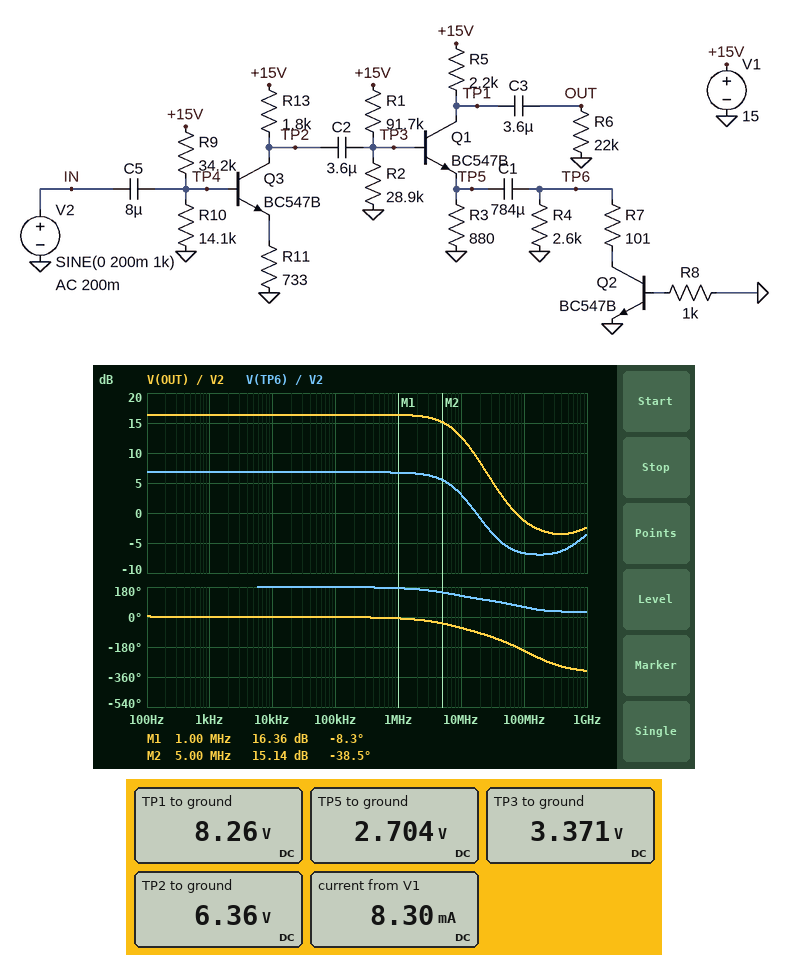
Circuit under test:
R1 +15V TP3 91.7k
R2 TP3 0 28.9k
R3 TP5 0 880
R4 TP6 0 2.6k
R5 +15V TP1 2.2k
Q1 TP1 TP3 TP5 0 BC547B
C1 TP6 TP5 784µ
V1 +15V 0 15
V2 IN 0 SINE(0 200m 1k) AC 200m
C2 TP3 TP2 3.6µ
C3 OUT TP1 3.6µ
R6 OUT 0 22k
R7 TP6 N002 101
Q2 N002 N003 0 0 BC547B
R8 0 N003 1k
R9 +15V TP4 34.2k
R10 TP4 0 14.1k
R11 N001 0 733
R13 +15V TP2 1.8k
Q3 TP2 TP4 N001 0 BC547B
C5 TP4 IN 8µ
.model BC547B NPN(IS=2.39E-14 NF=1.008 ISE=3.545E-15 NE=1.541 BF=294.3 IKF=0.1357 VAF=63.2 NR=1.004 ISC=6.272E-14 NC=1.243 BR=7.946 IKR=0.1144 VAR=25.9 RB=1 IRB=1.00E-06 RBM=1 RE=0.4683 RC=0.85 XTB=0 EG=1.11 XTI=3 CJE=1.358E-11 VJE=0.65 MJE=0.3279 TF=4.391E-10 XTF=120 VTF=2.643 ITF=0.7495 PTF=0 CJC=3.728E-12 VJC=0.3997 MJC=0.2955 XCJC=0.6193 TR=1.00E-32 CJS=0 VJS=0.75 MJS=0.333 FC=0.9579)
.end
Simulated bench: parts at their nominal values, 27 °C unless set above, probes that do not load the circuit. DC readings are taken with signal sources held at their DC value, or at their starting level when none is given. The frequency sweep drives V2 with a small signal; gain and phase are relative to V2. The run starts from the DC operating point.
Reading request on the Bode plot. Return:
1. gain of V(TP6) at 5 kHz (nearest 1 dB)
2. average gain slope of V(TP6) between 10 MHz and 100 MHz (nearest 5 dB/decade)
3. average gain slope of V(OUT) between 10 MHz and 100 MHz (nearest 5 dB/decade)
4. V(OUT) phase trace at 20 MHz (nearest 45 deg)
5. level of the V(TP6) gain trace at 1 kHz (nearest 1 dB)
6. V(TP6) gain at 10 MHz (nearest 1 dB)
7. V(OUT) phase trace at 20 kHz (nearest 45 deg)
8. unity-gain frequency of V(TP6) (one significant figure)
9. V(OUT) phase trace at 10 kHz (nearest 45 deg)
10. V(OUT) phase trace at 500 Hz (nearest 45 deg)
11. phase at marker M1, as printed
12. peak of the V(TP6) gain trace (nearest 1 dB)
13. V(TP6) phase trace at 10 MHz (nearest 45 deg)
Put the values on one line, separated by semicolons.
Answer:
7 dB; -10 dB/decade; -15 dB/decade; -90 deg; 7 dB; 3 dB; 0 deg; 20 MHz; 0 deg; 0 deg; -8.3 deg; 7 dB; 135 deg
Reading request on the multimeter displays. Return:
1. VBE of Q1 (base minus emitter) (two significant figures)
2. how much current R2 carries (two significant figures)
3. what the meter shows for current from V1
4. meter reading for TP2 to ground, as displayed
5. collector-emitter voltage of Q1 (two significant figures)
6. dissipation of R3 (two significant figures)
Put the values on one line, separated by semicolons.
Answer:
670 mV; 120 µA; 8.30 mA; 6.36 V; 5.6 V; 8.3 mW
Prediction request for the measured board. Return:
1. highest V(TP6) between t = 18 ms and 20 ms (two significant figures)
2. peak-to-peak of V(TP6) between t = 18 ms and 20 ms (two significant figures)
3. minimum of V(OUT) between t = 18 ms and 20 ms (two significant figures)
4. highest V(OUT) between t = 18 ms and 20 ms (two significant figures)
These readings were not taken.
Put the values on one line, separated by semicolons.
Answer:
440 mV; 870 mV; -1.3 V; 1.3 V
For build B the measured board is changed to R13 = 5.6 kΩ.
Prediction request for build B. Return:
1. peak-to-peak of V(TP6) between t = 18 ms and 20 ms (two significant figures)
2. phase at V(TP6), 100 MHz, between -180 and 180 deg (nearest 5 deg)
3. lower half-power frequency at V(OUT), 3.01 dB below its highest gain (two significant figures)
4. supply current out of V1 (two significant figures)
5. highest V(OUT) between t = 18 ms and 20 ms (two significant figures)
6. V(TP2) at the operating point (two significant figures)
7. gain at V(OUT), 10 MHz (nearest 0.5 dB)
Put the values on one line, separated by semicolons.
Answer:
510 mV; 0 deg; 37 Hz; 5.9 mA; 330 mV; 1.9 V; 8.0 dB
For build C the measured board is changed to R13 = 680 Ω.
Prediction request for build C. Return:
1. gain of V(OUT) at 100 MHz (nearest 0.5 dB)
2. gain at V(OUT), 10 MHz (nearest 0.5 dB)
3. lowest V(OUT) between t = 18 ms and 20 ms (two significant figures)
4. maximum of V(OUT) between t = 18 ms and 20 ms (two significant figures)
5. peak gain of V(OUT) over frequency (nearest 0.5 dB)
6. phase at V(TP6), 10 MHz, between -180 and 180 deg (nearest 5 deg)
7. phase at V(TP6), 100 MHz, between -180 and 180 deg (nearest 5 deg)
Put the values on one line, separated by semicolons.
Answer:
-3.0 dB; 7.5 dB; -530 mV; 530 mV; 8.5 dB; 150 deg; 75 deg
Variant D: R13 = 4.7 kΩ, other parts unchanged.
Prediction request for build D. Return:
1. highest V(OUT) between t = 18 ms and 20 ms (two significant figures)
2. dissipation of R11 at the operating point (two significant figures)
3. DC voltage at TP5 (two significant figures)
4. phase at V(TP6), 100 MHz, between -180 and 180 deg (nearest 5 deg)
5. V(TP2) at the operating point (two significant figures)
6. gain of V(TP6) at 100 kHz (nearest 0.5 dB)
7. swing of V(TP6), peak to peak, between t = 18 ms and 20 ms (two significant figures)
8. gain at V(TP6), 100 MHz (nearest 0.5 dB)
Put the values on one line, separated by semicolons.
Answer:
330 mV; 6.1 mW; 2.7 V; 0 deg; 2.2 V; -3.0 dB; 600 mV; -0.5 dB
